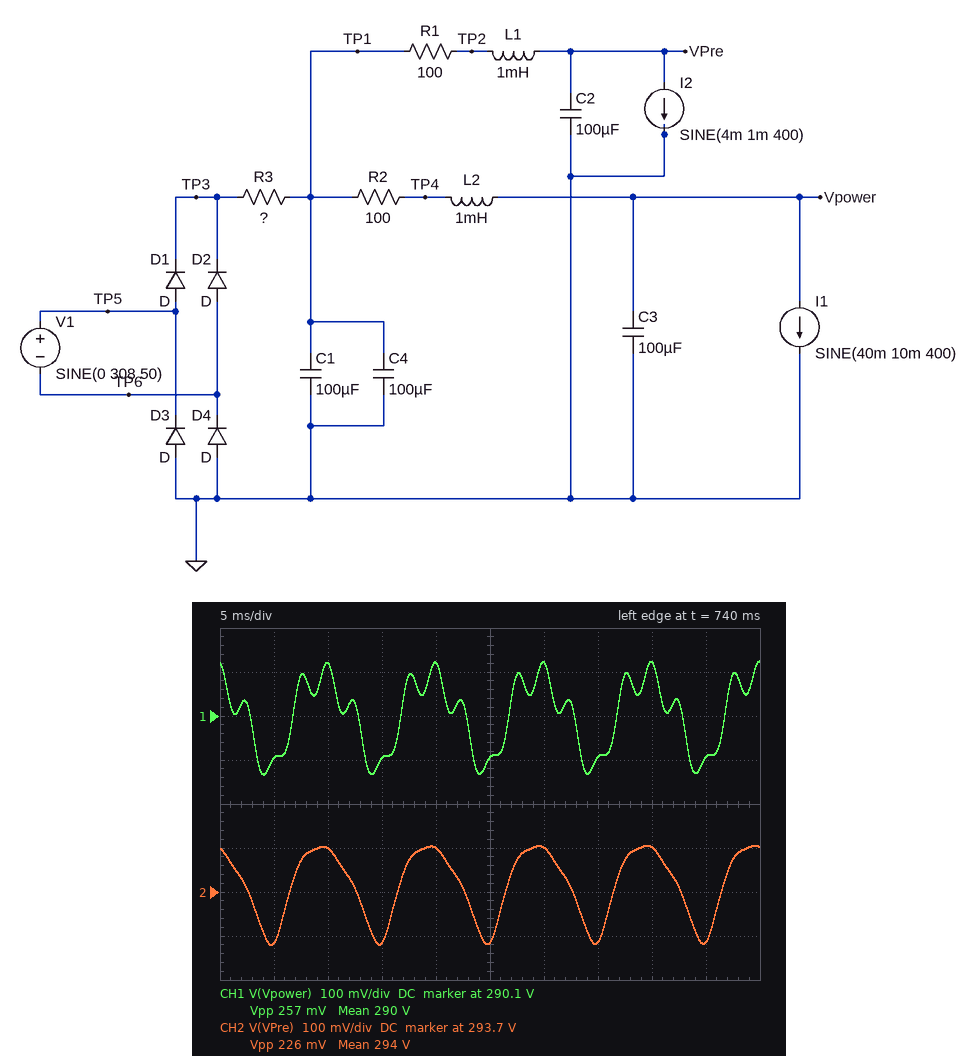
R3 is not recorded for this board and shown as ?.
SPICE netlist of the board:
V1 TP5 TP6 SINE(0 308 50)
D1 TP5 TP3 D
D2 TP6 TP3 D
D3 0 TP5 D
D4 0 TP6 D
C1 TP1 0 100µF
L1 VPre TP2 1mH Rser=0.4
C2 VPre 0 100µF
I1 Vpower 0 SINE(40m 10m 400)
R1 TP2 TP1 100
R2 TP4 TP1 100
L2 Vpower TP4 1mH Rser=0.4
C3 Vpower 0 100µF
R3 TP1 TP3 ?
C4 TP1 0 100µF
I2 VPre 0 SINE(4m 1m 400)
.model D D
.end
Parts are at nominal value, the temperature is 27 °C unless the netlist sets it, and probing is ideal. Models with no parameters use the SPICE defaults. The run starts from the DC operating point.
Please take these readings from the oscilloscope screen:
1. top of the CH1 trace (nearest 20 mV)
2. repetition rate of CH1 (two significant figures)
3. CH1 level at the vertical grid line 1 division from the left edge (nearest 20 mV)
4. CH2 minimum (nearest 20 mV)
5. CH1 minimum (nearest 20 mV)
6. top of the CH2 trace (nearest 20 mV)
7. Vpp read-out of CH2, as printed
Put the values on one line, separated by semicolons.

290.22 V; 100 Hz; 290.00 V; 293.58 V; 289.96 V; 293.80 V; 226 mV
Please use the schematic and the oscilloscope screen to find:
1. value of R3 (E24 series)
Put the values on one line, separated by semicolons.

33 Ω
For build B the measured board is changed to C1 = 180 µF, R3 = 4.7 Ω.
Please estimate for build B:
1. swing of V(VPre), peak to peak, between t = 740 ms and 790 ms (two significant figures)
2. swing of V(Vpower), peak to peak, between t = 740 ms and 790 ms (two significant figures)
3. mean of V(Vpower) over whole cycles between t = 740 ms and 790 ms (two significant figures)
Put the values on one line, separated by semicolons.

170 mV; 200 mV; 300 V
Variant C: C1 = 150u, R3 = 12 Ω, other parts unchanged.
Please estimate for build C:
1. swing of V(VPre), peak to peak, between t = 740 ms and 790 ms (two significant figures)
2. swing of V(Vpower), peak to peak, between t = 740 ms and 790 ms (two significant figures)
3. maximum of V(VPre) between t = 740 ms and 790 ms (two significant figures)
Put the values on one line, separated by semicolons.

190 mV; 220 mV; 300 V
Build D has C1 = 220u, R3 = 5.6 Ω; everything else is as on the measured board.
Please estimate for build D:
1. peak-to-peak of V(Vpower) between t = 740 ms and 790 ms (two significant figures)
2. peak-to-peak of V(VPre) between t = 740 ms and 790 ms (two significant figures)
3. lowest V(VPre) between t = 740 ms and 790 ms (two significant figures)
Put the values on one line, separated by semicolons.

190 mV; 150 mV; 300 V
